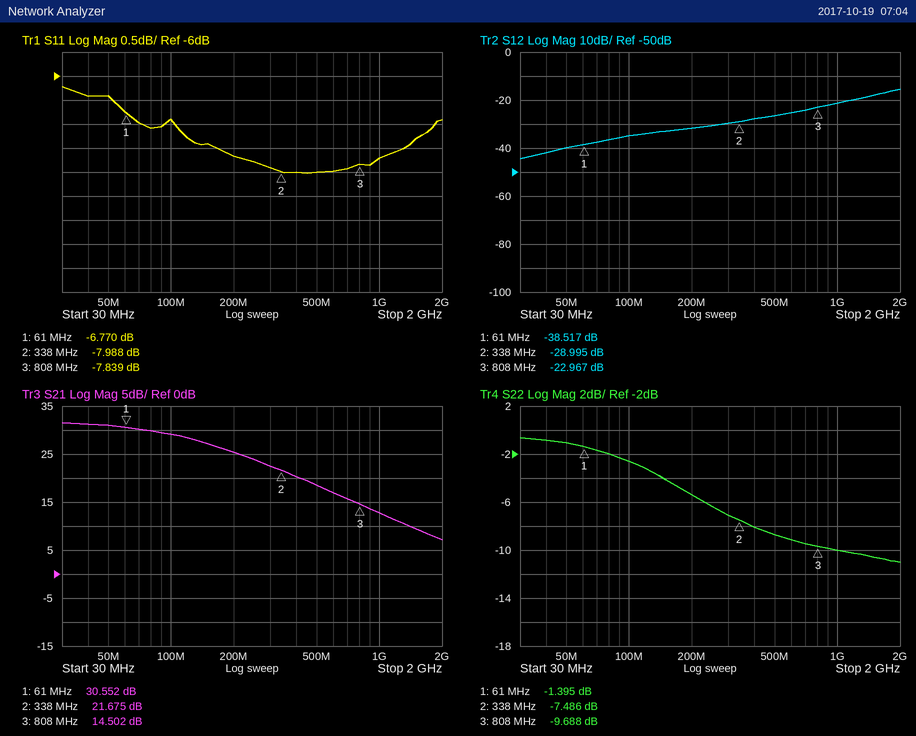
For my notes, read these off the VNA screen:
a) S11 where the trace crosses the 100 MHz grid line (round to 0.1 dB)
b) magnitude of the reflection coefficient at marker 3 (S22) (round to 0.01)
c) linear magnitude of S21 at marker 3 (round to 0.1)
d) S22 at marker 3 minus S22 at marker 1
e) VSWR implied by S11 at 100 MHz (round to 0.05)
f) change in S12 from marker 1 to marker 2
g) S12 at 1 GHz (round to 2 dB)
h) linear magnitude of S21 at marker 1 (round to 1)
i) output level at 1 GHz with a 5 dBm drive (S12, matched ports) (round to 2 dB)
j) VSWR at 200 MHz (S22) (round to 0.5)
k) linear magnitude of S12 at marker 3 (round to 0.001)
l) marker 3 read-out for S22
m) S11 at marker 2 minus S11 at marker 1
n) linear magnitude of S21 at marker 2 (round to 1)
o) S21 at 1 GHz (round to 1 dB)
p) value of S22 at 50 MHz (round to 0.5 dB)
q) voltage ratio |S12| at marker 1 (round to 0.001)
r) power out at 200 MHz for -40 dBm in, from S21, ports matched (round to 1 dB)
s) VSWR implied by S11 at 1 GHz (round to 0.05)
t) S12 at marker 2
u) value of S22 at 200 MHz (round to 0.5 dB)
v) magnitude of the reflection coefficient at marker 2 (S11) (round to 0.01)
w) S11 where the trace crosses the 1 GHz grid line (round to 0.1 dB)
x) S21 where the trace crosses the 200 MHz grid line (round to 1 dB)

-6.9 dB
0.33
5.3
-8.293 dB
2.65
9.522 dB
-22 dB
34
-16 dBm
3.5
0.071
-9.688 dB
-1.218 dB
12
13 dB
-1.0 dB
0.012
-15 dBm
2.40
-28.995 dB
-5.5 dB
0.40
-7.7 dB
25 dB
